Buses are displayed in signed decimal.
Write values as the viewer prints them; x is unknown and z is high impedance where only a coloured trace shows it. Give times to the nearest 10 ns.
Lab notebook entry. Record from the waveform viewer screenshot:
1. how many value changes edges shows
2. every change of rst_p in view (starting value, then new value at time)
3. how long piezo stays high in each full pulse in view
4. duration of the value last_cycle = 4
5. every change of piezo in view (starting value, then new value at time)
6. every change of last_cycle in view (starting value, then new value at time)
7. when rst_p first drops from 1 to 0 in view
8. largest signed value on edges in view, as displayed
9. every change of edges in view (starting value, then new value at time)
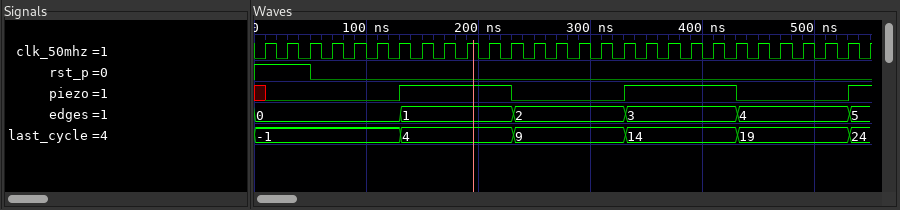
5
1, 0 at 50 ns
100 ns, 100 ns
100 ns
x, 0 at 10 ns, 1 at 130 ns, 0 at 230 ns, 1 at 330 ns, 0 at 430 ns, 1 at 530 ns
-1, 4 at 130 ns, 9 at 230 ns, 14 at 330 ns, 19 at 430 ns, 24 at 530 ns
50 ns
5
0, 1 at 130 ns, 2 at 230 ns, 3 at 330 ns, 4 at 430 ns, 5 at 530 ns
